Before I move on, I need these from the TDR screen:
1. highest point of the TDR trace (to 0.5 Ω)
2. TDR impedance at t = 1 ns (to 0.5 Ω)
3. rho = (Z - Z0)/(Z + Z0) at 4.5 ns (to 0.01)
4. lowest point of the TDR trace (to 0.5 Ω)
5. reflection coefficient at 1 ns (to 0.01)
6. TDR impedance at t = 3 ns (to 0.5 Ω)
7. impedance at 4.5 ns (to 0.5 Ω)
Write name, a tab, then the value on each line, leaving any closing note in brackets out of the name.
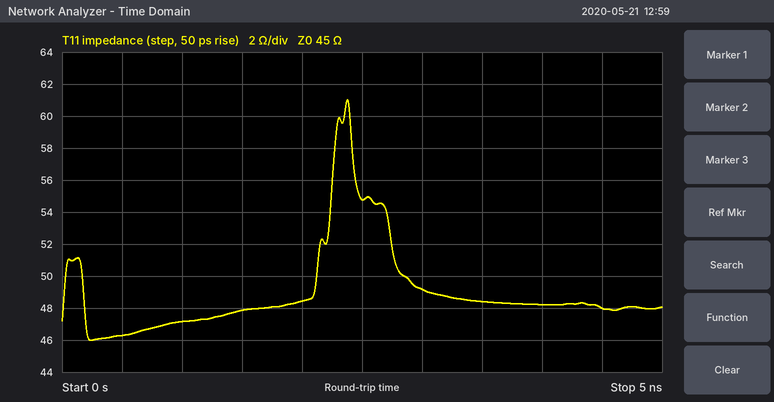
highest point of the TDR trace	61.0 Ω
TDR impedance at t = 1 ns	47.0 Ω
rho = (Z - Z0)/(Z + Z0) at 4.5 ns	+0.03
lowest point of the TDR trace	46.0 Ω
reflection coefficient at 1 ns	+0.02
TDR impedance at t = 3 ns	49.0 Ω
impedance at 4.5 ns	48.0 Ω
